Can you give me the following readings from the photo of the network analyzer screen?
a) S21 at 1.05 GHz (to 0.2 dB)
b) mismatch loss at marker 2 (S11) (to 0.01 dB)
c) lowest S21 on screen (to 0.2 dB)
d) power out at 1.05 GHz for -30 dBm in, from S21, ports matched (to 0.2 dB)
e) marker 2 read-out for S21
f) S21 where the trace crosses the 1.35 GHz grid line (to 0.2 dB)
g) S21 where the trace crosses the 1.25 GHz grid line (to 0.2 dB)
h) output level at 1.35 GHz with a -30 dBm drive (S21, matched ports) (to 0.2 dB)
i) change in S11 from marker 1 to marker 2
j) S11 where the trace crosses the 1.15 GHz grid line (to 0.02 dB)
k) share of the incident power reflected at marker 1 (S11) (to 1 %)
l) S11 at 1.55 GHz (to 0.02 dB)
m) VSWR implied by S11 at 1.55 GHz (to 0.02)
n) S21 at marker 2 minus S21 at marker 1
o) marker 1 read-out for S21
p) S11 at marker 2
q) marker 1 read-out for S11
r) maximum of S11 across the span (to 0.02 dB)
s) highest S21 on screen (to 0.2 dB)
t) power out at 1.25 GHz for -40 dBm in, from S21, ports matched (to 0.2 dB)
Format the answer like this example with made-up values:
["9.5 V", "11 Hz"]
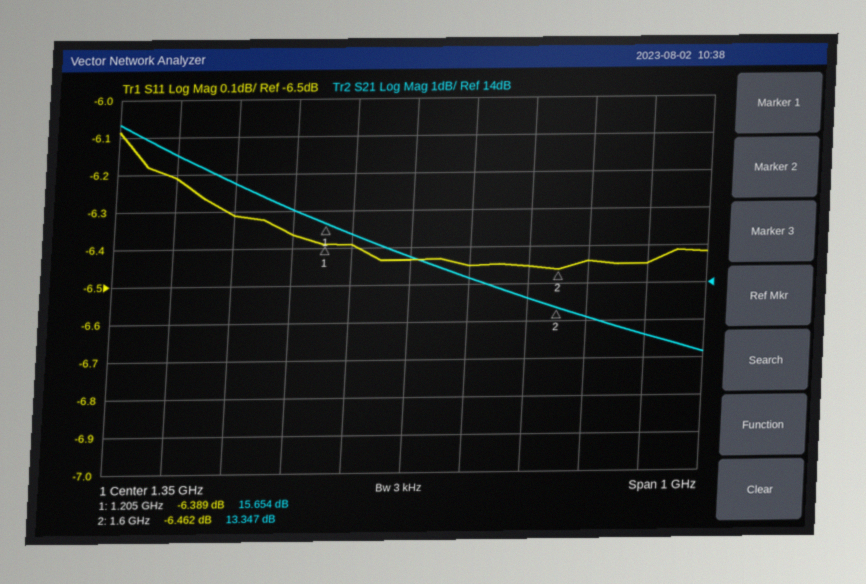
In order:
["16.8 dB", "1.11 dB", "12.2 dB", "-13.2 dBm", "13.347 dB", "14.8 dB", "15.4 dB", "-15.2 dBm", "-0.073 dB", "-6.36 dB", "23 %", "-6.46 dB", "2.82", "-2.307 dB", "15.654 dB", "-6.462 dB", "-6.389 dB", "-6.08 dB", "18.4 dB", "-24.6 dBm"]
